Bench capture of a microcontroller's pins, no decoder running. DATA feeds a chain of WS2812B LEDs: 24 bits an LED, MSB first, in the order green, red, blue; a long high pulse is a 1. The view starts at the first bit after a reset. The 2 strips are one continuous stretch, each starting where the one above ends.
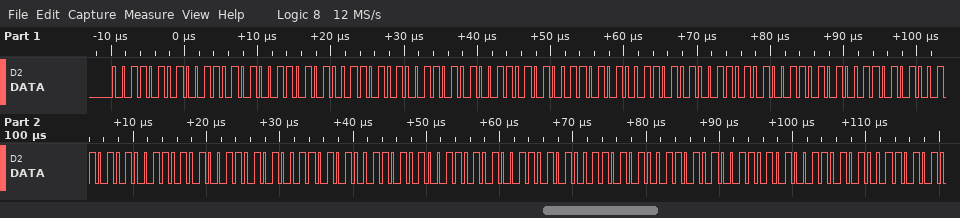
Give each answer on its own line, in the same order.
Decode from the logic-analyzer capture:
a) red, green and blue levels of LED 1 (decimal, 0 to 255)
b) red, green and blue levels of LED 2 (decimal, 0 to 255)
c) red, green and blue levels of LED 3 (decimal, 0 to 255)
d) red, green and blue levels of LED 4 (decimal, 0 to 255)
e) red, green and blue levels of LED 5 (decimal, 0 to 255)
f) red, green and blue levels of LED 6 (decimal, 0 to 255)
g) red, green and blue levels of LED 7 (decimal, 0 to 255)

53, 53, 53
53, 53, 53
53, 53, 53
53, 53, 53
53, 53, 53
53, 53, 53
53, 53, 53
